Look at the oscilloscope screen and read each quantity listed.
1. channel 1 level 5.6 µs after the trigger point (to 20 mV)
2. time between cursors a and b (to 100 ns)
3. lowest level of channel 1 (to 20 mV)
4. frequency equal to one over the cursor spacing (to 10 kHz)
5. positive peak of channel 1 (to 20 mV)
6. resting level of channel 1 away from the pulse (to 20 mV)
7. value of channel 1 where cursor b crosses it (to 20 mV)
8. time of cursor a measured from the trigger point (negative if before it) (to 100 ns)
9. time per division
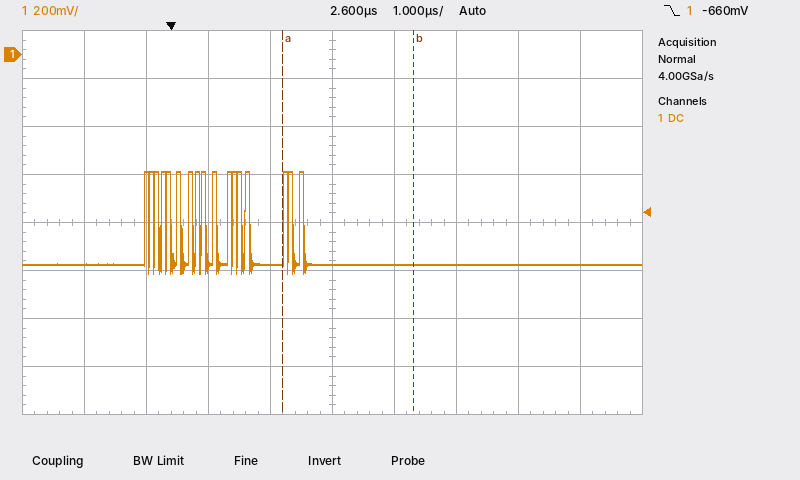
-880 mV
2.1 µs
-920 mV
480 kHz
-480 mV
-880 mV
-880 mV
+1.8 µs
1 µs
